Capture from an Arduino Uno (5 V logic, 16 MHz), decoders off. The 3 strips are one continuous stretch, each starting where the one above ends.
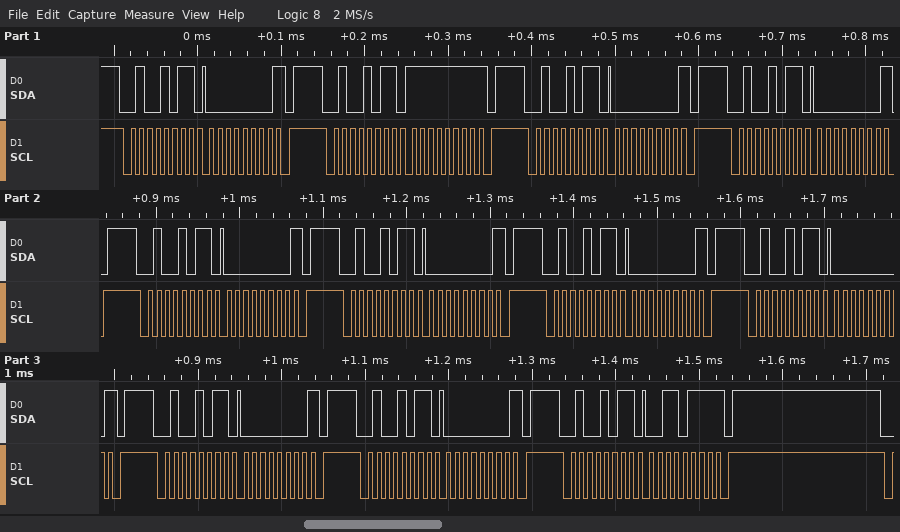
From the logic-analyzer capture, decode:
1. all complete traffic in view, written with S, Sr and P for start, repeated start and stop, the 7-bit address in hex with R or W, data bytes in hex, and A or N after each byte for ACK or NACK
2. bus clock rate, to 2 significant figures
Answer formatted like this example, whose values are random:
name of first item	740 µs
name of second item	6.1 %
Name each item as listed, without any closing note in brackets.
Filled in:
all complete traffic in view, written with S, Sr and P for start, repeated start and stop, the 7-bit address in hex with R or W, data bytes in hex, and A or N after each byte for ACK or NACK	S 25R A 00 N P S 25R A FF N P S 25R A 00 N P S 25R A 00 N P S 25R A 00 N P S 25R A 00 N P S 25R A 00 N P S 25R A 00 N P S 25R A 00 N P S 25R A 00 N P S 25R A 37 N P
bus clock rate, to 2 significant figures	100 kHz
